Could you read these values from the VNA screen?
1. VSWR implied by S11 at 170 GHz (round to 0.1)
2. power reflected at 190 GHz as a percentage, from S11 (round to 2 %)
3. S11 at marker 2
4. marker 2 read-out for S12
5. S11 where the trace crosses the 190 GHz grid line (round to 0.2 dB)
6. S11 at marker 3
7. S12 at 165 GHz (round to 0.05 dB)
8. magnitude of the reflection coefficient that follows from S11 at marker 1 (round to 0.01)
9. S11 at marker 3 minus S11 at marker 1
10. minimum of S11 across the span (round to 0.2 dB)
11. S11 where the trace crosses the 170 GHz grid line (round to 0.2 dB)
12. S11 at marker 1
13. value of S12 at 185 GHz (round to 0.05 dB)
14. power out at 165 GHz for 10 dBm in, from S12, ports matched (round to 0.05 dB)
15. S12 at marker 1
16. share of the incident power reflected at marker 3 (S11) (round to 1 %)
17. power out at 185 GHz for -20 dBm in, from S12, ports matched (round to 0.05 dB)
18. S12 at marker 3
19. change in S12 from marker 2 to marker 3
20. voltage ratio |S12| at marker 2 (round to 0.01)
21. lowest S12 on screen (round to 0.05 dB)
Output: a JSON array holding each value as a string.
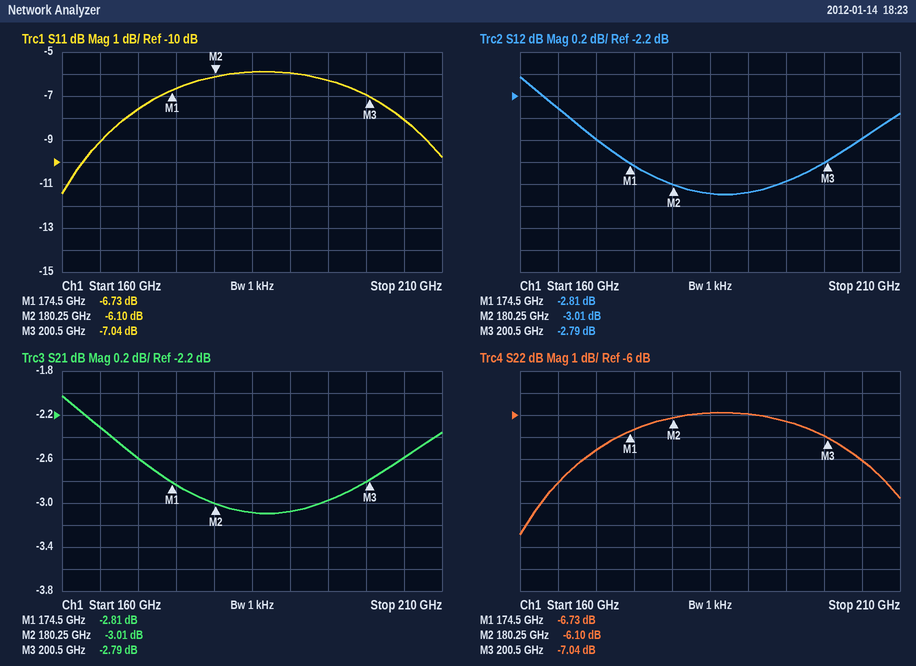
["2.4", "26 %", "-6.10 dB", "-3.01 dB", "-6.0 dB", "-7.04 dB", "-2.30 dB", "0.46", "-0.31 dB", "-11.4 dB", "-7.6 dB", "-6.73 dB", "-3.10 dB", "7.70 dBm", "-2.81 dB", "20 %", "-23.10 dBm", "-2.79 dB", "0.22 dB", "0.71", "-3.10 dB"]
